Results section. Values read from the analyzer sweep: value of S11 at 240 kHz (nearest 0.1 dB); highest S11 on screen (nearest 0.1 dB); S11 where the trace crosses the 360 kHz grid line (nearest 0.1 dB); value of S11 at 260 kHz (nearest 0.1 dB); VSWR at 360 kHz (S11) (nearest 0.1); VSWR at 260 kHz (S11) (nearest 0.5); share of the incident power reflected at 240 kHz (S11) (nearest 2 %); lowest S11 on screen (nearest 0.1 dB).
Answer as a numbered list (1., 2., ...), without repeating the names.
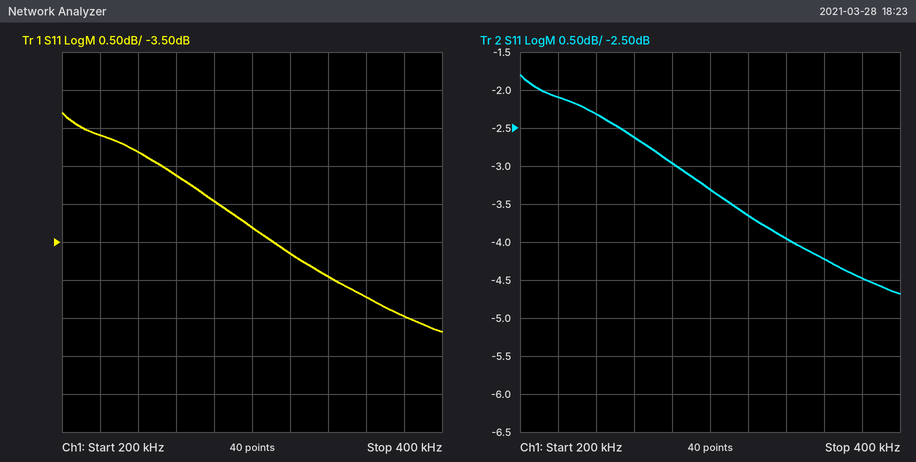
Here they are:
1. -2.3 dB
2. -1.8 dB
3. -4.2 dB
4. -2.6 dB
5. 4.2
6. 6.5
7. 58 %
8. -4.7 dB
